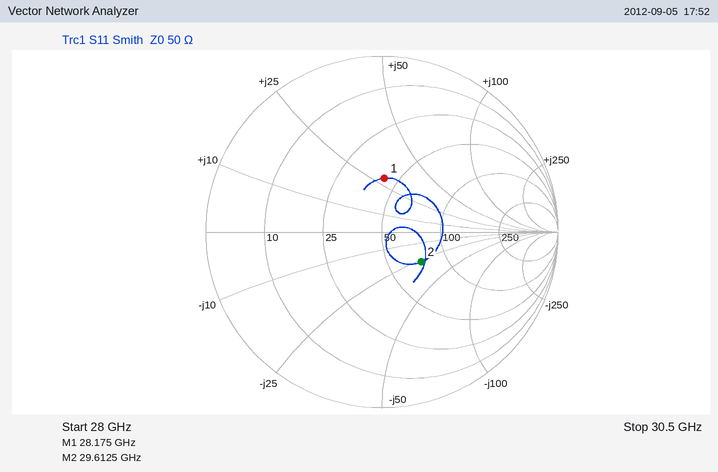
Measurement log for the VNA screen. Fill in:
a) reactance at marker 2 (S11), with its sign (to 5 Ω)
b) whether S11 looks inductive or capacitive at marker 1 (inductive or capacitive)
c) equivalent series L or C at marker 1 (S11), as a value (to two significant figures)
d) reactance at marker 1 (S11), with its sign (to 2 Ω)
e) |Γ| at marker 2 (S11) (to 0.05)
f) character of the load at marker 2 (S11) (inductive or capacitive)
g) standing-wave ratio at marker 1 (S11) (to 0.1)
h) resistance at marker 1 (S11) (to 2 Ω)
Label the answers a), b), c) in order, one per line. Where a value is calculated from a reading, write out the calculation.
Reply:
a) -25 Ω
b) inductive
c) L = 28 Ω/(2π × 28.175 GHz) ≈ 158 pH, so 160 pH to two significant figures
d) +28 Ω
e) 0.30
f) capacitive
g) 1.9
h) 42 Ω
